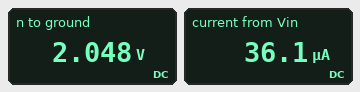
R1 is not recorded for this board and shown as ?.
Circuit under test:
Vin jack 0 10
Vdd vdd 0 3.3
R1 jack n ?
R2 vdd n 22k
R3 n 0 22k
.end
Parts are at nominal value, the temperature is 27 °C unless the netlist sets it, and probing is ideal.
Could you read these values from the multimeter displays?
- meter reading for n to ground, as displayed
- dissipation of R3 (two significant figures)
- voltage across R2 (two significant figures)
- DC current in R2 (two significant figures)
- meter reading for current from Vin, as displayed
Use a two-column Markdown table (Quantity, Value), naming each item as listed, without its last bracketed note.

| Quantity | Value |
|---|---|
| meter reading for n to ground, as displayed | 2.048 V |
| dissipation of R3 | 190 µW |
| voltage across R2 | 1.3 V |
| DC current in R2 | 57 µA |
| meter reading for current from Vin, as displayed | 36.1 µA |
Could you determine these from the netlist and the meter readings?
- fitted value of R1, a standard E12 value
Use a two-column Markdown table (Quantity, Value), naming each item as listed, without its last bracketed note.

| Quantity | Value |
|---|---|
| fitted value of R1, a standard E12 value | 220 kΩ |
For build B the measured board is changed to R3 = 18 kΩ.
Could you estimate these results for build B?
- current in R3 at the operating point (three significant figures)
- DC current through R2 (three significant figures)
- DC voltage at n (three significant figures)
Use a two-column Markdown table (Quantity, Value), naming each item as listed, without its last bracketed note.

| Quantity | Value |
|---|---|
| current in R3 at the operating point | 103 µA |
| DC current through R2 | 65.8 µA |
| DC voltage at n | 1.85 V |
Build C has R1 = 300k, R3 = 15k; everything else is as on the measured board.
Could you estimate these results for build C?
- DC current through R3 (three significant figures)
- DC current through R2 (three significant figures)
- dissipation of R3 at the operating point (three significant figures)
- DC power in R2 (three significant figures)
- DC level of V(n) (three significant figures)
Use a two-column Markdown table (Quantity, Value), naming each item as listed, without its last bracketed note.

| Quantity | Value |
|---|---|
| DC current through R3 | 106 µA |
| DC current through R2 | 77.8 µA |
| dissipation of R3 at the operating point | 168 µW |
| DC power in R2 | 133 µW |
| DC level of V(n) | 1.59 V |
